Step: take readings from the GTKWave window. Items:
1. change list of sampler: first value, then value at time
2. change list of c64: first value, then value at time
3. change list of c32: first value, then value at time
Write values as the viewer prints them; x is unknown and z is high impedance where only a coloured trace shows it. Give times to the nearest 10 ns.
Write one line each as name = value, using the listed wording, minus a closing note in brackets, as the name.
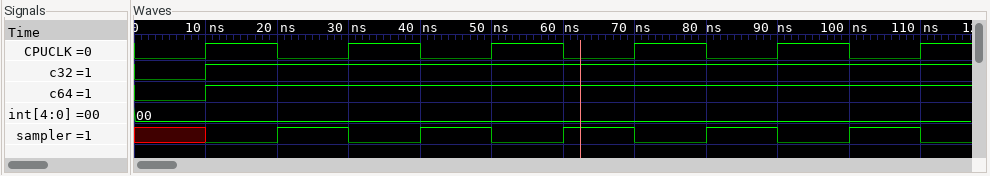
change list of sampler: first value, then value at time = x, 0 at 10 ns, 1 at 20 ns, 0 at 30 ns, 1 at 40 ns, 0 at 50 ns, 1 at 60 ns, 0 at 70 ns, 1 at 80 ns, 0 at 90 ns, 1 at 100 ns, 0 at 110 ns
change list of c64: first value, then value at time = 0, 1 at 10 ns
change list of c32: first value, then value at time = 0, 1 at 10 ns
